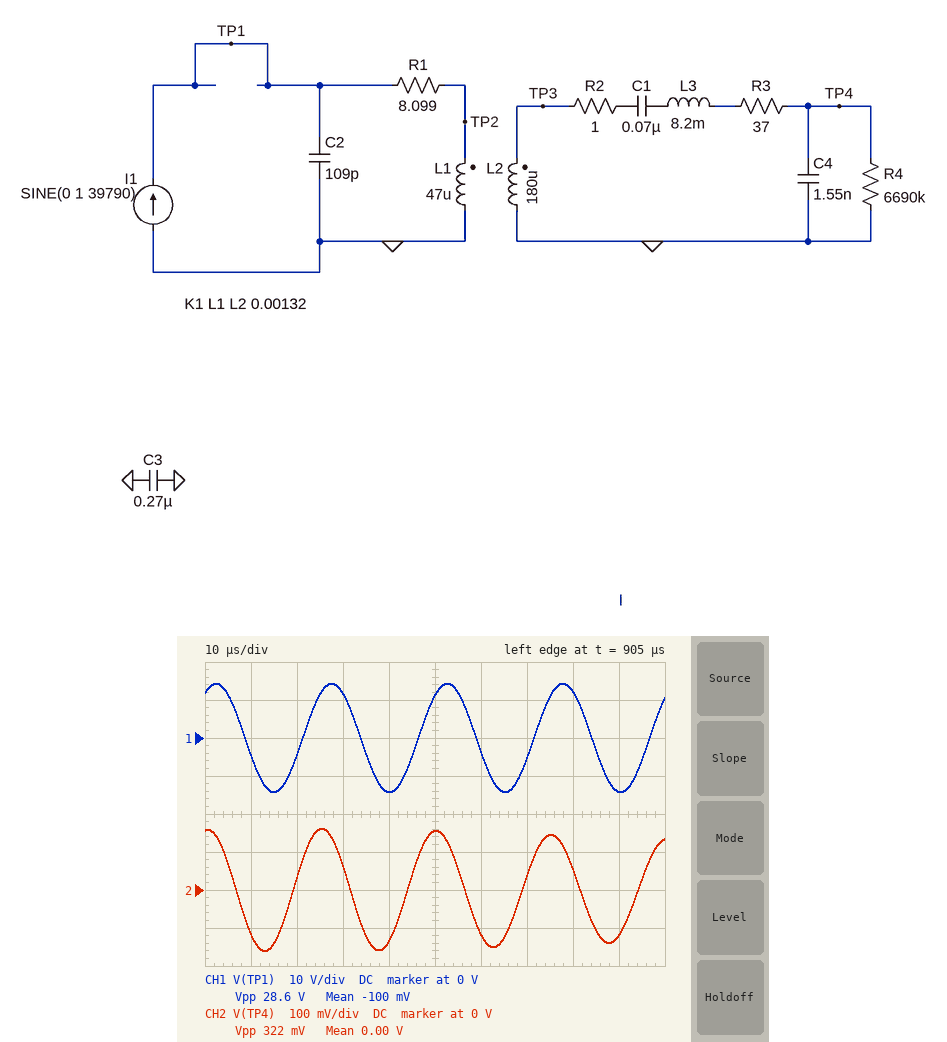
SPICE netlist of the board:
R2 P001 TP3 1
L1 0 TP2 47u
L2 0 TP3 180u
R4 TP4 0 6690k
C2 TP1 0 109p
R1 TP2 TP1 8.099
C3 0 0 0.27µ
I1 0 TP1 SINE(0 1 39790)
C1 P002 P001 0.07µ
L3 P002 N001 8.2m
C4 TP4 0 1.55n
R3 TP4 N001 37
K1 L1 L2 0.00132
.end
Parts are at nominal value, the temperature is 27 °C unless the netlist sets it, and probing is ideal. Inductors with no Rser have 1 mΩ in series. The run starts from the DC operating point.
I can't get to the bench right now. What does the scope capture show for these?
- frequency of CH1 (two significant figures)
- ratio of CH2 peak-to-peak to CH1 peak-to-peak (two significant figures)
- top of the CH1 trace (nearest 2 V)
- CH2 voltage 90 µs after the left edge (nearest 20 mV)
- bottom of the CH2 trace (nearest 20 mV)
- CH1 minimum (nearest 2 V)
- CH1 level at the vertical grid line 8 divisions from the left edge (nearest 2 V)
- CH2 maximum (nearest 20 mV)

40 kHz
0.011
14 V
-120 mV
-160 mV
-14 V
12 V
160 mV
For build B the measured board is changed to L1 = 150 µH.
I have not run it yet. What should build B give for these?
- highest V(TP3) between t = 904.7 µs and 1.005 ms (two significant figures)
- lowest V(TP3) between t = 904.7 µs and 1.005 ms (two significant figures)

59 mV
-59 mV
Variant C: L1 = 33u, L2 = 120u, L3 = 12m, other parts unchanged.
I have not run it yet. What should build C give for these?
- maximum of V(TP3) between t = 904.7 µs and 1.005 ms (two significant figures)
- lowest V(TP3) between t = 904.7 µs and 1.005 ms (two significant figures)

19 mV
-19 mV
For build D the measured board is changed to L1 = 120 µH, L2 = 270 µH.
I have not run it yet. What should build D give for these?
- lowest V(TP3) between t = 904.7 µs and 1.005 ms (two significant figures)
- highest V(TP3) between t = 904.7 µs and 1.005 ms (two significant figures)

-68 mV
68 mV
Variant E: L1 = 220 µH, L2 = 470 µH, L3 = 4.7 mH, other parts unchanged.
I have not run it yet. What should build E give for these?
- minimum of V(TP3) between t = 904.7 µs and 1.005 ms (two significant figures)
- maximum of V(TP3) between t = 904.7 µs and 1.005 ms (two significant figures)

-120 mV
120 mV
